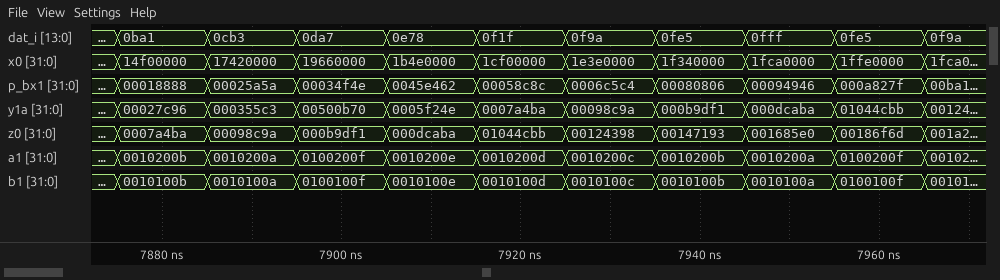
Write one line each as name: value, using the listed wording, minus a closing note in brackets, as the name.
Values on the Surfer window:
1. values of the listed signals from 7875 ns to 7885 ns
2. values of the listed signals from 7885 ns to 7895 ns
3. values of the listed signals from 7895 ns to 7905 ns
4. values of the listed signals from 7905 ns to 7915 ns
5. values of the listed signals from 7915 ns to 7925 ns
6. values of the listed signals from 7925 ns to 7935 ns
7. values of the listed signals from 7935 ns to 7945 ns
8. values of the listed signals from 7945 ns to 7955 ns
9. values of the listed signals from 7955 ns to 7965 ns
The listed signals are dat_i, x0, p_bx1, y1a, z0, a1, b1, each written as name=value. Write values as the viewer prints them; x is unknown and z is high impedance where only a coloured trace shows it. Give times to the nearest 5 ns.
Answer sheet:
values of the listed signals from 7875 ns to 7885 ns: dat_i=0ba1, x0=14f00000, p_bx1=00018888, y1a=00027c96, z0=0007a4ba, a1=0010200b, b1=0010100b
values of the listed signals from 7885 ns to 7895 ns: dat_i=0cb3, x0=17420000, p_bx1=00025a5a, y1a=000355c3, z0=00098c9a, a1=0010200a, b1=0010100a
values of the listed signals from 7895 ns to 7905 ns: dat_i=0da7, x0=19660000, p_bx1=00034f4e, y1a=00500b70, z0=000b9df1, a1=0100200f, b1=0100100f
values of the listed signals from 7905 ns to 7915 ns: dat_i=0e78, x0=1b4e0000, p_bx1=0045e462, y1a=0005f24e, z0=000dcaba, a1=0010200e, b1=0010100e
values of the listed signals from 7915 ns to 7925 ns: dat_i=0f1f, x0=1cf00000, p_bx1=00058c8c, y1a=0007a4ba, z0=01044cbb, a1=0010200d, b1=0010100d
values of the listed signals from 7925 ns to 7935 ns: dat_i=0f9a, x0=1e3e0000, p_bx1=0006c5c4, y1a=00098c9a, z0=00124398, a1=0010200c, b1=0010100c
values of the listed signals from 7935 ns to 7945 ns: dat_i=0fe5, x0=1f340000, p_bx1=00080806, y1a=000b9df1, z0=00147193, a1=0010200b, b1=0010100b
values of the listed signals from 7945 ns to 7955 ns: dat_i=0fff, x0=1fca0000, p_bx1=00094946, y1a=000dcaba, z0=001685e0, a1=0010200a, b1=0010100a
values of the listed signals from 7955 ns to 7965 ns: dat_i=0fe5, x0=1ffe0000, p_bx1=000a827f, y1a=01044cbb, z0=00186f6d, a1=0100200f, b1=0100100f
